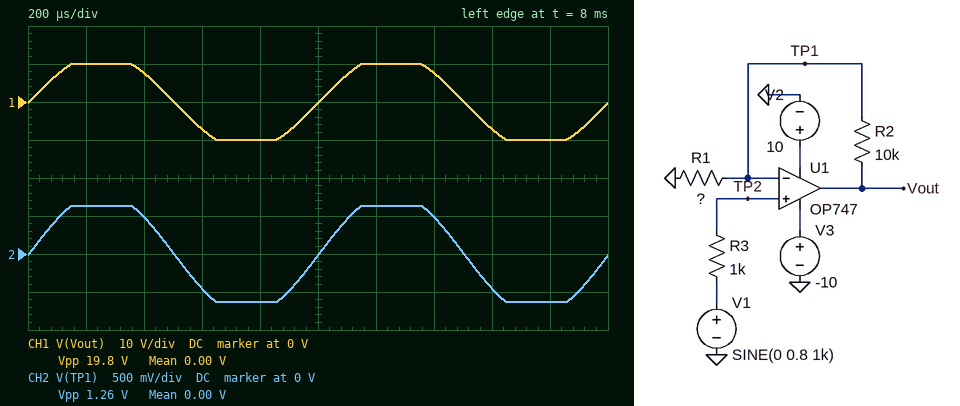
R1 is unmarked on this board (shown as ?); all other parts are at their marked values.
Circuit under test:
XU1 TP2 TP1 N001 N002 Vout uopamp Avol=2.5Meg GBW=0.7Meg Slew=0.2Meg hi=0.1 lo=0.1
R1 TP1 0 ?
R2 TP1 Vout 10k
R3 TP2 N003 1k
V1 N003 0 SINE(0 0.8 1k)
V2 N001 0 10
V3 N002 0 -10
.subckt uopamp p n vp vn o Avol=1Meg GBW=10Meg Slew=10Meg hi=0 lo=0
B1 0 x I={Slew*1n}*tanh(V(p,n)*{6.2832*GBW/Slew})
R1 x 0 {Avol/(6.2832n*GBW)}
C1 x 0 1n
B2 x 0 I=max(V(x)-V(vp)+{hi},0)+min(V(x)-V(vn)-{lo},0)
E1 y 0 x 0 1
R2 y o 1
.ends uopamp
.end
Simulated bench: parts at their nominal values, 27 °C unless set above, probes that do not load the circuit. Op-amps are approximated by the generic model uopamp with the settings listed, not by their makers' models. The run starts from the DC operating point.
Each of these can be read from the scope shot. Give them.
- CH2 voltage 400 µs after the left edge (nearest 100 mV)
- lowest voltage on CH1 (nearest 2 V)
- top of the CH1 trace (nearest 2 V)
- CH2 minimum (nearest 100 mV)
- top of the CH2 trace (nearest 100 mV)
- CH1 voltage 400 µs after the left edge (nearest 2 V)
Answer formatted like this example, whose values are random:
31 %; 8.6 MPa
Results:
500 mV; -10 V; 10 V; -600 mV; 600 mV; 8 V
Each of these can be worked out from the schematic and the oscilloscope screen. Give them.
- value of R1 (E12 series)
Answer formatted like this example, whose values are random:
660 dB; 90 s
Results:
680 Ω
